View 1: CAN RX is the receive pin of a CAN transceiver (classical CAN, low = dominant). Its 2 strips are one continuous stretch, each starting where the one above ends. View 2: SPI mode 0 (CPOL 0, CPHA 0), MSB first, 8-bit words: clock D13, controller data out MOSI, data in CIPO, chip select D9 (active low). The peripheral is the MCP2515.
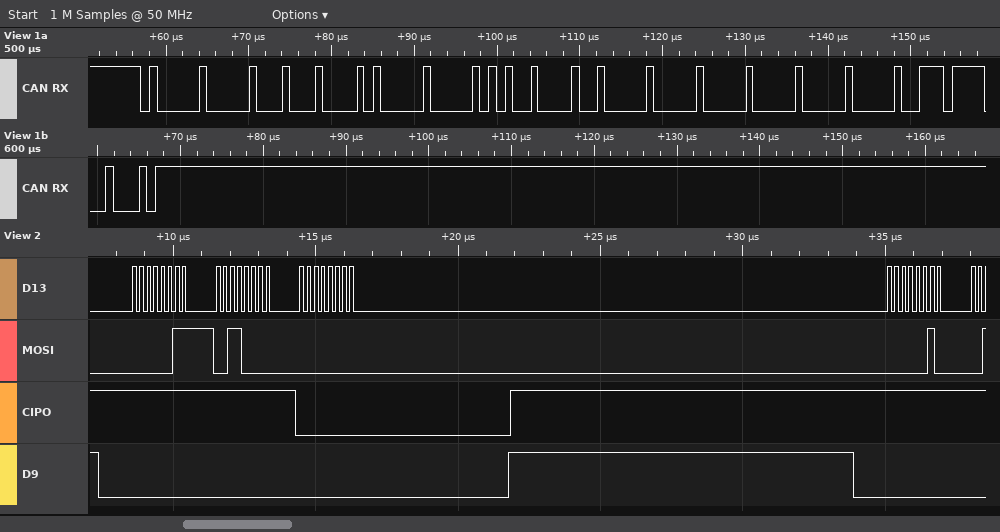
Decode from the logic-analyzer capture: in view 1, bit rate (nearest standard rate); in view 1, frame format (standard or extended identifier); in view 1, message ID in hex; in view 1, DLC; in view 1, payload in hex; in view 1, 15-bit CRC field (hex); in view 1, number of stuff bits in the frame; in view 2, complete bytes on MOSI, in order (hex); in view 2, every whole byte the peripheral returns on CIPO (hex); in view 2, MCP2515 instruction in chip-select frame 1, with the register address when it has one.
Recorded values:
1000 kbit/s
standard
0x400
8
85 00 14 84 80 00 00 00
0x3BC8
10
03 30 00 02
FF FF 00 FF
READ 0x30
